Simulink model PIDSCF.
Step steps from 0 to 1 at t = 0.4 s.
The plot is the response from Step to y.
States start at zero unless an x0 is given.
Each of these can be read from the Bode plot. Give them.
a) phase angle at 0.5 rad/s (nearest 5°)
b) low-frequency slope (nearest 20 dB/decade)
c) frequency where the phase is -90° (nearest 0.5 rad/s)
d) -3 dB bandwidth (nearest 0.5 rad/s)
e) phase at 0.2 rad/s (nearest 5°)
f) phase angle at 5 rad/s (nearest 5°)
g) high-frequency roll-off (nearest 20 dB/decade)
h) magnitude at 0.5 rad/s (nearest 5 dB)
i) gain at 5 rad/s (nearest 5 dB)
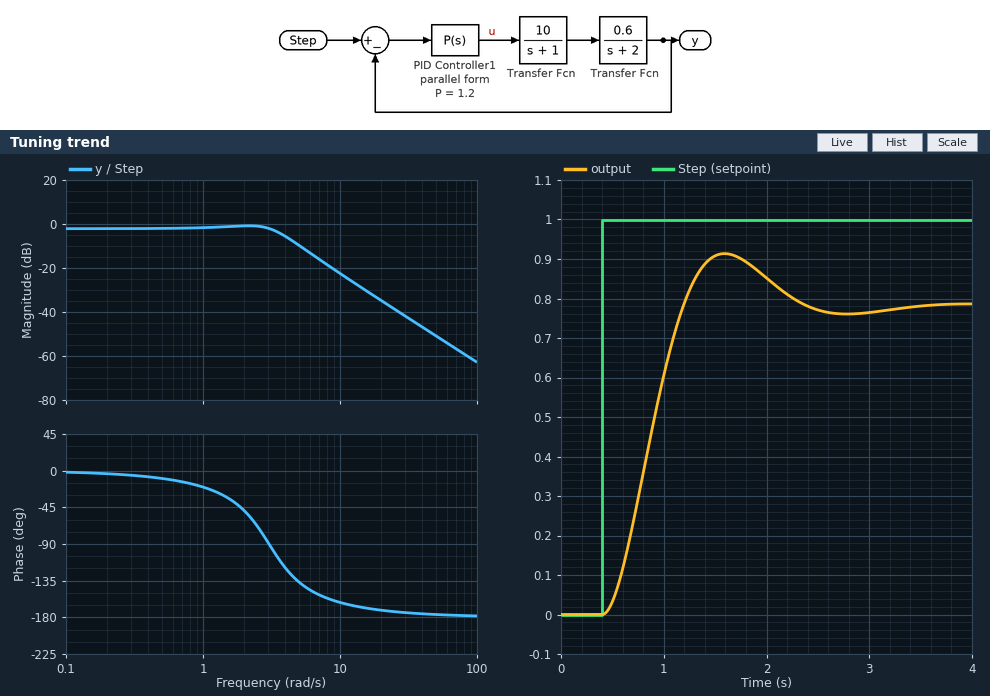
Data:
-10°
0 dB/decade
3.0 rad/s
4.0 rad/s
-5°
-135°
-40 dB/decade
0 dB
-10 dB
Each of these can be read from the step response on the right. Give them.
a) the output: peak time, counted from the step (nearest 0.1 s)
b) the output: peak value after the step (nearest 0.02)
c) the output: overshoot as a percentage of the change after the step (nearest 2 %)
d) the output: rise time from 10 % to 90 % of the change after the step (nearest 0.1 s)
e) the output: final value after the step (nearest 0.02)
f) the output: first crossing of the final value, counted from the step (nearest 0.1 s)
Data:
1.2 s
0.92
16 %
0.5 s
0.78
0.8 s
